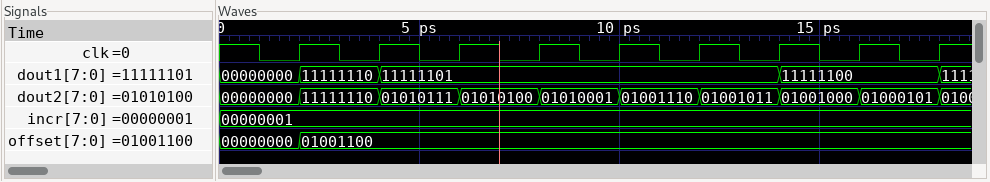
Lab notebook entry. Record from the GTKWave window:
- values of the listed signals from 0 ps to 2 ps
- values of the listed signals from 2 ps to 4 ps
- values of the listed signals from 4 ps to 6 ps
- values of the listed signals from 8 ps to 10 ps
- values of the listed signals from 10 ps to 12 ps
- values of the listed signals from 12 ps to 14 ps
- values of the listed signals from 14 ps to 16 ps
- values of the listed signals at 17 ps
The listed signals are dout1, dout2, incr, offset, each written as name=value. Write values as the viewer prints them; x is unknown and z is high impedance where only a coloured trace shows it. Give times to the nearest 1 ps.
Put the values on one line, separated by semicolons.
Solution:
dout1=00000000, dout2=00000000, incr=00000001, offset=00000000; dout1=11111110, dout2=11111110, incr=00000001, offset=01001100; dout1=11111101, dout2=01010111, incr=00000001, offset=01001100; dout1=11111101, dout2=01010001, incr=00000001, offset=01001100; dout1=11111101, dout2=01001110, incr=00000001, offset=01001100; dout1=11111101, dout2=01001011, incr=00000001, offset=01001100; dout1=11111100, dout2=01001000, incr=00000001, offset=01001100; dout1=11111100, dout2=01000101, incr=00000001, offset=01001100
